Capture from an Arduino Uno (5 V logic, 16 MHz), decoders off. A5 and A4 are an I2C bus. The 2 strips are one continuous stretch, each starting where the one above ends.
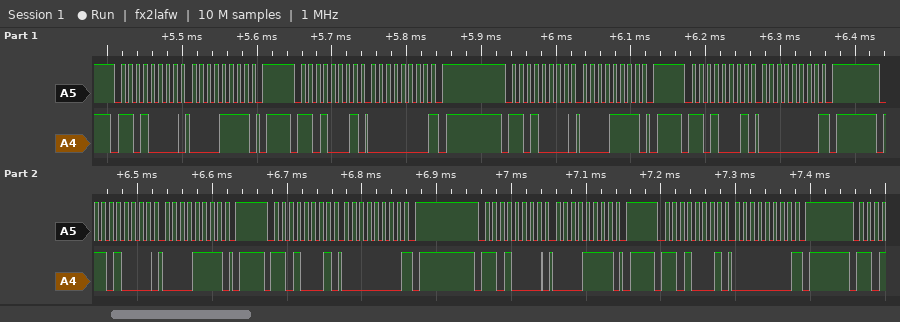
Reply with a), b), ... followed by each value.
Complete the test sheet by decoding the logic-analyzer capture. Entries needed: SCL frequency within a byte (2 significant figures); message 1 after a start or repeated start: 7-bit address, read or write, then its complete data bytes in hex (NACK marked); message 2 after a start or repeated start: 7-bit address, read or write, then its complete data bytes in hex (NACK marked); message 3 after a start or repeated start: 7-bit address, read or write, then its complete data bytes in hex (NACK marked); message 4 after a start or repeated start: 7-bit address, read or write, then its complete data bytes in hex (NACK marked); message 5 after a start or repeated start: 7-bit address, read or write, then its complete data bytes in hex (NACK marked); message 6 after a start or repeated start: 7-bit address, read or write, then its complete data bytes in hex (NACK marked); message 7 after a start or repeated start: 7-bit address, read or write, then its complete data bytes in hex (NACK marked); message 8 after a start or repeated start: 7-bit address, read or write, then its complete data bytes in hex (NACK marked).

a) 100 kHz
b) 0x68 write: 0F
c) 0x68 read: 00 NACK
d) 0x68 write: 0F
e) 0x68 read: 00 NACK
f) 0x68 write: 0F
g) 0x68 read: 00 NACK
h) 0x68 write: 0F
i) 0x68 read: 00 NACK
